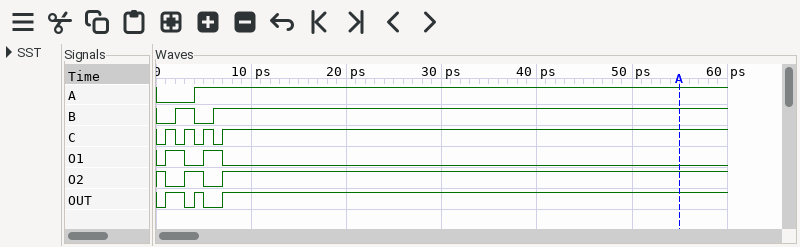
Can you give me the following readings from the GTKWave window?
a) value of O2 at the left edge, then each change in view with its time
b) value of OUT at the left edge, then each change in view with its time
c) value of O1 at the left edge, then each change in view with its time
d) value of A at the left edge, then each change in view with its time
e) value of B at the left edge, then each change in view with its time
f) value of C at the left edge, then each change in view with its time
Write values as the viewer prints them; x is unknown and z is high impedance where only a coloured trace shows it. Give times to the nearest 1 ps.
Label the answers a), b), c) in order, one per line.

a) 1, 0 at 1 ps, 1 at 3 ps, 0 at 5 ps, 1 at 7 ps
b) 0, 1 at 1 ps, 0 at 3 ps, 1 at 4 ps, 0 at 5 ps, 1 at 7 ps
c) 0, 1 at 1 ps, 0 at 3 ps, 1 at 5 ps, 0 at 7 ps
d) 0, 1 at 4 ps
e) 0, 1 at 2 ps, 0 at 4 ps, 1 at 6 ps
f) 0, 1 at 1 ps, 0 at 2 ps, 1 at 3 ps, 0 at 4 ps, 1 at 5 ps, 0 at 6 ps, 1 at 7 ps
